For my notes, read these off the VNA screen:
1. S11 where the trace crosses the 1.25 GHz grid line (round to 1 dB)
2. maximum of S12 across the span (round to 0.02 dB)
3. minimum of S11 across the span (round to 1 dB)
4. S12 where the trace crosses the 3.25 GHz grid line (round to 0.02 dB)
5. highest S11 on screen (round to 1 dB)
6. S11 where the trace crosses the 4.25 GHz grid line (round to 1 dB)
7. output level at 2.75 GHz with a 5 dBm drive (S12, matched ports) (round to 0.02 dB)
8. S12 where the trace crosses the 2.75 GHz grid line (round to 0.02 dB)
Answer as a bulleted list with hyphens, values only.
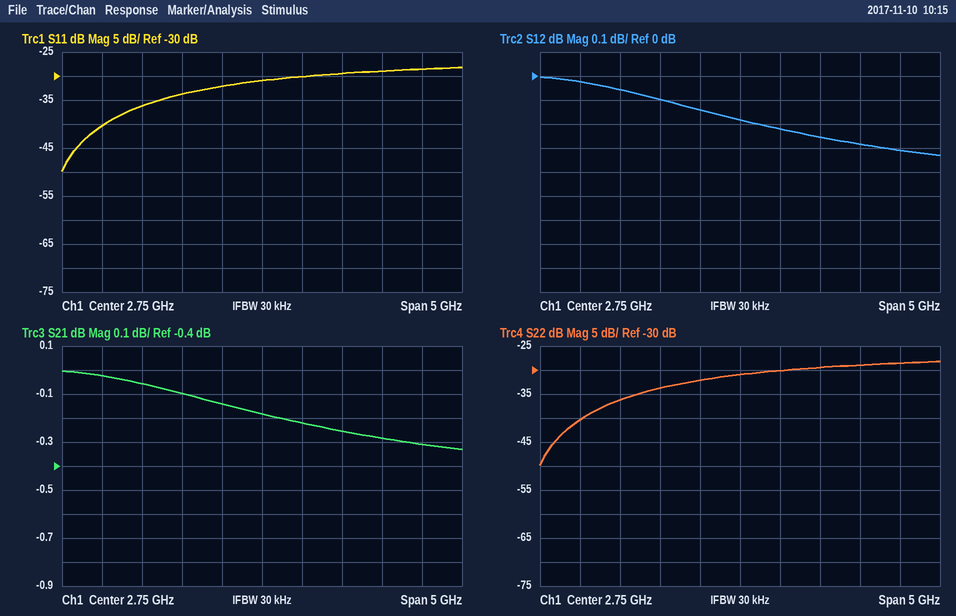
- -36 dB
- 0.00 dB
- -50 dB
- -0.22 dB
- -28 dB
- -29 dB
- 4.82 dBm
- -0.18 dB
